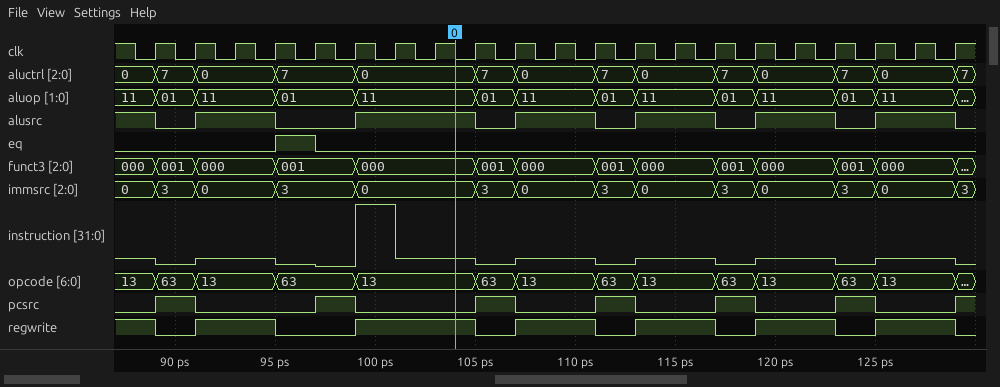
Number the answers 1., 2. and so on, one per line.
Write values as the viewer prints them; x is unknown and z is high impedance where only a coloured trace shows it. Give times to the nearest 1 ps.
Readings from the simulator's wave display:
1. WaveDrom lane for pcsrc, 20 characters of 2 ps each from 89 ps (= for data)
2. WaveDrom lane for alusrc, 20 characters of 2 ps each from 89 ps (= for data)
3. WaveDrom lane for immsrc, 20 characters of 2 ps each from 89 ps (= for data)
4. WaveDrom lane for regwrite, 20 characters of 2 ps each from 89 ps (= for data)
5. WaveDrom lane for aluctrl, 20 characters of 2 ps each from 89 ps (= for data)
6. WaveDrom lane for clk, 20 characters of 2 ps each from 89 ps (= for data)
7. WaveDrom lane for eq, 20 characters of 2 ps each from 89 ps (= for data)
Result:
1. {name: 'pcsrc', wave: '10..10..10.10.10.10.'}
2. {name: 'alusrc', wave: '01.0.1..01.01.01.01.'}
3. {name: 'immsrc', wave: '==.=.=..==.==.==.==.', data: '3 0 3 0 3 0 3 0 3 0 3 0'}
4. {name: 'regwrite', wave: '01.0.1..01.01.01.01.'}
5. {name: 'aluctrl', wave: '==.=.=..==.==.==.==.', data: '7 0 7 0 7 0 7 0 7 0 7 0'}
6. {name: 'clk', wave: 'p...................'}
7. {name: 'eq', wave: '0..10...............'}
